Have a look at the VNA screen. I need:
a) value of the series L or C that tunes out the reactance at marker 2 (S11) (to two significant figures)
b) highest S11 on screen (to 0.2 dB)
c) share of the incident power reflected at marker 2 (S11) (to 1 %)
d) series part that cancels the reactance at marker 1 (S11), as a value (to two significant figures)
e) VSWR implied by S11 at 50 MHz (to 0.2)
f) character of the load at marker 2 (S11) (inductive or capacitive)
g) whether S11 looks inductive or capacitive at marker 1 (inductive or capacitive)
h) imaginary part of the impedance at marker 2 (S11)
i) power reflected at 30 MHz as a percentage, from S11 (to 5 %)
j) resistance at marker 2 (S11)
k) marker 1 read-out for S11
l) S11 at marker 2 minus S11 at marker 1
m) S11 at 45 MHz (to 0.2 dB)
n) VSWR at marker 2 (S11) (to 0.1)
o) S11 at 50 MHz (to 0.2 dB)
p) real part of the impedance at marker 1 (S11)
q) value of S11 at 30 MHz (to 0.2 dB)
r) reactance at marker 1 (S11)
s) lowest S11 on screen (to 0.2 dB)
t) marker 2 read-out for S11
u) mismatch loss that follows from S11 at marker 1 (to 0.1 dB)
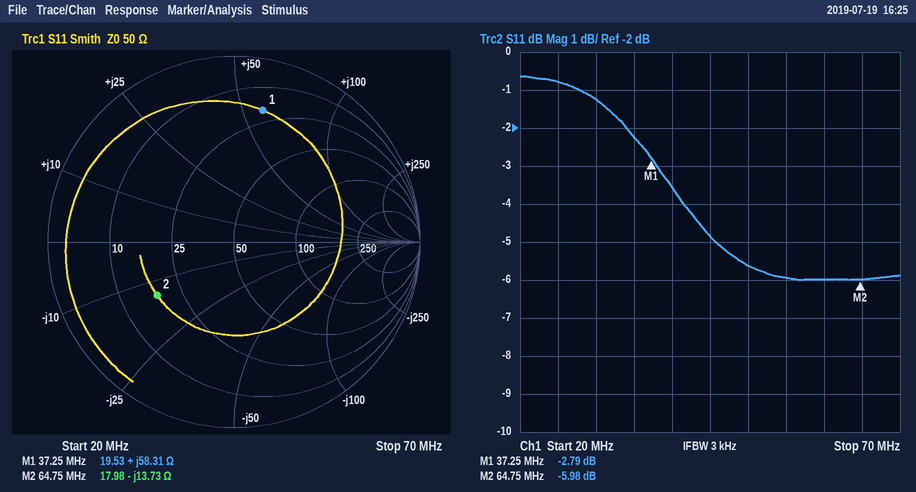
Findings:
34 nH
-0.6 dB
25 %
73 pF
3.2
capacitive
inductive
-13.73 Ω
75 %
17.98 Ω
-2.79 dB
-3.19 dB
-4.8 dB
3.0
-5.6 dB
19.53 Ω
-1.2 dB
+58.31 Ω
-6.0 dB
-5.98 dB
3.2 dB
